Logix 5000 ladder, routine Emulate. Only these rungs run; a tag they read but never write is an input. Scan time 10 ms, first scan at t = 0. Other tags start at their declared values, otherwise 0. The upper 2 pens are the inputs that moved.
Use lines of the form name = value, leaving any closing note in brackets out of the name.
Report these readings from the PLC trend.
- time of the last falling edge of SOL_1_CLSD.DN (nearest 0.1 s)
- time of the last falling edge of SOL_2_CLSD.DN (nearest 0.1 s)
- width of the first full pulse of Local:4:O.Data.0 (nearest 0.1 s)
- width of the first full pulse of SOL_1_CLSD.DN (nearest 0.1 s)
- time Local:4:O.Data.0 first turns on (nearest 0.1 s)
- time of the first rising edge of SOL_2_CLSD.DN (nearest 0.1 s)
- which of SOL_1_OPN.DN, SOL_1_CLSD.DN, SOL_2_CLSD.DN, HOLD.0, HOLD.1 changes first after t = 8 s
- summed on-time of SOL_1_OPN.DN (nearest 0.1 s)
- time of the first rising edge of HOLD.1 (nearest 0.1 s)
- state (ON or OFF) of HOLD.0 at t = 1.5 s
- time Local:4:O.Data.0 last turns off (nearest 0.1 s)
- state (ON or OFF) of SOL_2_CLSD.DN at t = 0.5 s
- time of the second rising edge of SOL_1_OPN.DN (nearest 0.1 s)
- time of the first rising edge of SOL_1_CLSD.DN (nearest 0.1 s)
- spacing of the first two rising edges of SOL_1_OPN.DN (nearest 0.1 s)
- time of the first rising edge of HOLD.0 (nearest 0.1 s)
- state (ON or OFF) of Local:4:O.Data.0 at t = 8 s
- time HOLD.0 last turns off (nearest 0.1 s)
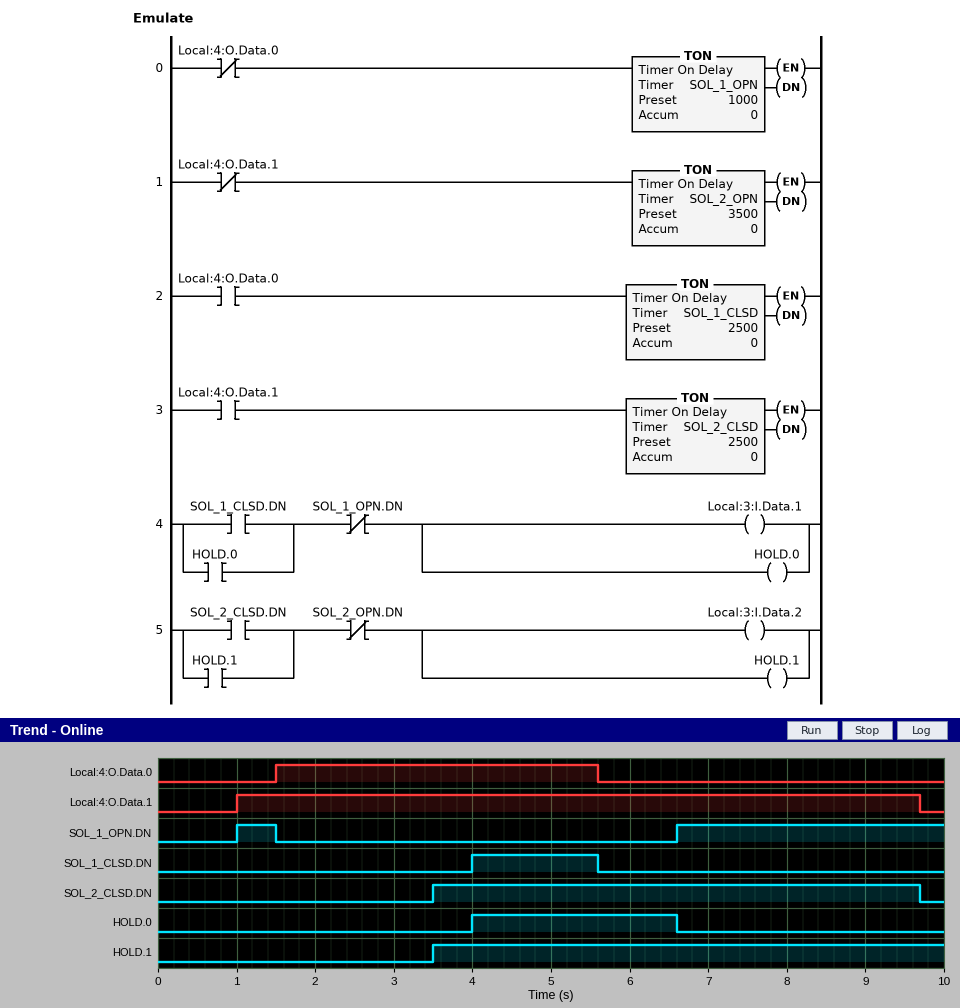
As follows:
time of the last falling edge of SOL_1_CLSD.DN = 5.6 s
time of the last falling edge of SOL_2_CLSD.DN = 9.7 s
width of the first full pulse of Local:4:O.Data.0 = 4.1 s
width of the first full pulse of SOL_1_CLSD.DN = 1.6 s
time Local:4:O.Data.0 first turns on = 1.5 s
time of the first rising edge of SOL_2_CLSD.DN = 3.5 s
which of SOL_1_OPN.DN, SOL_1_CLSD.DN, SOL_2_CLSD.DN, HOLD.0, HOLD.1 changes first after t = 8 s = SOL_2_CLSD.DN
summed on-time of SOL_1_OPN.DN = 3.9 s
time of the first rising edge of HOLD.1 = 3.5 s
state (ON or OFF) of HOLD.0 at t = 1.5 s = OFF
time Local:4:O.Data.0 last turns off = 5.6 s
state (ON or OFF) of SOL_2_CLSD.DN at t = 0.5 s = OFF
time of the second rising edge of SOL_1_OPN.DN = 6.6 s
time of the first rising edge of SOL_1_CLSD.DN = 4.0 s
spacing of the first two rising edges of SOL_1_OPN.DN = 5.6 s
time of the first rising edge of HOLD.0 = 4.0 s
state (ON or OFF) of Local:4:O.Data.0 at t = 8 s = OFF
time HOLD.0 last turns off = 6.6 s
